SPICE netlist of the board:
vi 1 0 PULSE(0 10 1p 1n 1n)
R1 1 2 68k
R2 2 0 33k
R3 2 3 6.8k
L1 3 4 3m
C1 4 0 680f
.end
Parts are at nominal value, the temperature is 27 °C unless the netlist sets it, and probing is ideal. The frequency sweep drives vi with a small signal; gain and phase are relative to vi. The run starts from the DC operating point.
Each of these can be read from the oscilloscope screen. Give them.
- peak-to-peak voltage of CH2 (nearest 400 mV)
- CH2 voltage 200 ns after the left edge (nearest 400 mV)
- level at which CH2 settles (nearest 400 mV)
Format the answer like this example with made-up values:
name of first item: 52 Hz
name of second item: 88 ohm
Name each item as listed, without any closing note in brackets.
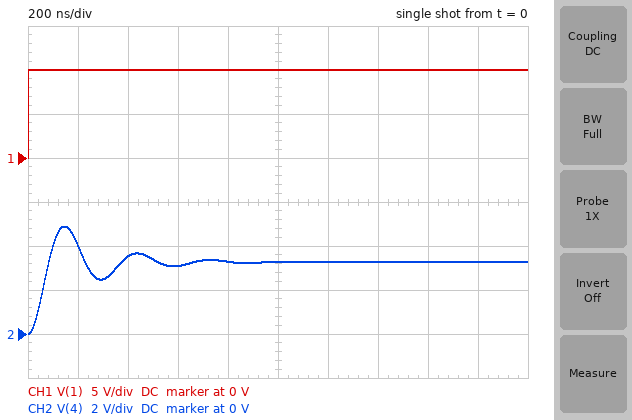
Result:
peak-to-peak voltage of CH2: 4.8 V
CH2 voltage 200 ns after the left edge: 4.0 V
level at which CH2 settles: 3.2 V
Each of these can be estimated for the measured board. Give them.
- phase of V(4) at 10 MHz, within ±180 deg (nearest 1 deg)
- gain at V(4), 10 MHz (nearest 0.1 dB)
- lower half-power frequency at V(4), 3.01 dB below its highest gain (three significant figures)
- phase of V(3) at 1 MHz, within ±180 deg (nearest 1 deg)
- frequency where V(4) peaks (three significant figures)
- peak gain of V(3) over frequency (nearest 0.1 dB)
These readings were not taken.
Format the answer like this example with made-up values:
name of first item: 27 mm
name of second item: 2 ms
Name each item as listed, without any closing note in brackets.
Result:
phase of V(4) at 10 MHz, within ±180 deg: -170 deg
gain at V(4), 10 MHz: -26.8 dB
lower half-power frequency at V(4), 3.01 dB below its highest gain: 2.44 MHz
phase of V(3) at 1 MHz, within ±180 deg: -8 deg
frequency where V(4) peaks: 3.35 MHz
peak gain of V(3) over frequency: -9.7 dB
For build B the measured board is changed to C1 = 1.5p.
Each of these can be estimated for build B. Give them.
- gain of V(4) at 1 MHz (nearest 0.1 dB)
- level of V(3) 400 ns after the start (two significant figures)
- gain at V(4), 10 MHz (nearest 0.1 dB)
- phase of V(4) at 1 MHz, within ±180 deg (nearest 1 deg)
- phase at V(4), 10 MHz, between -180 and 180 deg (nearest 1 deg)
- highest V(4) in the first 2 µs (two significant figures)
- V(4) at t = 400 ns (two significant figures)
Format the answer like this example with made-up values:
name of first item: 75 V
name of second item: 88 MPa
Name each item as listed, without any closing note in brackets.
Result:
gain of V(4) at 1 MHz: -8.5 dB
level of V(3) 400 ns after the start: 3.5 V
gain at V(4), 10 MHz: -34.3 dB
phase of V(4) at 1 MHz, within ±180 deg: -18 deg
phase at V(4), 10 MHz, between -180 and 180 deg: -171 deg
highest V(4) in the first 2 µs: 4.4 V
V(4) at t = 400 ns: 3.0 V
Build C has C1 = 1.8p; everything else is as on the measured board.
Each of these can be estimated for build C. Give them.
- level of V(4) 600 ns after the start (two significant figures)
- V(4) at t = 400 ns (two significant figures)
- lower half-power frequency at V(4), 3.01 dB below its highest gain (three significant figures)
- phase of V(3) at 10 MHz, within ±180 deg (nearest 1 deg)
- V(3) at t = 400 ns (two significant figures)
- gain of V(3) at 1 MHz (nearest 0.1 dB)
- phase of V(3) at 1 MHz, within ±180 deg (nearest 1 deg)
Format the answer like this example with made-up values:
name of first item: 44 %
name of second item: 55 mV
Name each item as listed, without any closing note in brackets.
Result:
level of V(4) 600 ns after the start: 3.2 V
V(4) at t = 400 ns: 3.3 V
lower half-power frequency at V(4), 3.01 dB below its highest gain: 624 kHz
phase of V(3) at 10 MHz, within ±180 deg: 9 deg
V(3) at t = 400 ns: 3.6 V
gain of V(3) at 1 MHz: -10.4 dB
phase of V(3) at 1 MHz, within ±180 deg: -23 deg
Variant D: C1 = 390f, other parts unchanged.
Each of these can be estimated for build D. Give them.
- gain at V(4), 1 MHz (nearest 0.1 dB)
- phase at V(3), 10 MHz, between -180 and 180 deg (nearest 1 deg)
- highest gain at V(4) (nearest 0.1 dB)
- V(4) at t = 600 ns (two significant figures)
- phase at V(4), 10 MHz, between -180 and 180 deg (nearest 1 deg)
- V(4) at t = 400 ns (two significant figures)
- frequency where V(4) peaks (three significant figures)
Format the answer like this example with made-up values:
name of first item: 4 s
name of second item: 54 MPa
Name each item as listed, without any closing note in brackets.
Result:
gain at V(4), 1 MHz: -9.3 dB
phase at V(3), 10 MHz, between -180 and 180 deg: 11 deg
highest gain at V(4): 0 dB
V(4) at t = 600 ns: 3.3 V
phase at V(4), 10 MHz, between -180 and 180 deg: -169 deg
V(4) at t = 400 ns: 3.1 V
frequency where V(4) peaks: 4.52 MHz
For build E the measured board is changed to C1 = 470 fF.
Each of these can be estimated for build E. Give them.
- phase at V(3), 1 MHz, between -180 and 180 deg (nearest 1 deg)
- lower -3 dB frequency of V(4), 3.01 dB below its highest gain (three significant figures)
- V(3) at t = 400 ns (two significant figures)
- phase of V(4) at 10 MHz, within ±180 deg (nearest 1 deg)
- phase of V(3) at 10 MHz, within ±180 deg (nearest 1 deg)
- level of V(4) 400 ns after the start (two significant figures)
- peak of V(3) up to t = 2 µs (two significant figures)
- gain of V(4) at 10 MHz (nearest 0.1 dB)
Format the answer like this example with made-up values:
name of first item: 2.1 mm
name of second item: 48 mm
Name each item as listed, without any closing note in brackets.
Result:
phase at V(3), 1 MHz, between -180 and 180 deg: -5 deg
lower -3 dB frequency of V(4), 3.01 dB below its highest gain: 3.22 MHz
V(3) at t = 400 ns: 3.4 V
phase of V(4) at 10 MHz, within ±180 deg: -169 deg
phase of V(3) at 10 MHz, within ±180 deg: 11 deg
level of V(4) 400 ns after the start: 3.6 V
peak of V(3) up to t = 2 µs: 3.8 V
gain of V(4) at 10 MHz: -23.1 dB
